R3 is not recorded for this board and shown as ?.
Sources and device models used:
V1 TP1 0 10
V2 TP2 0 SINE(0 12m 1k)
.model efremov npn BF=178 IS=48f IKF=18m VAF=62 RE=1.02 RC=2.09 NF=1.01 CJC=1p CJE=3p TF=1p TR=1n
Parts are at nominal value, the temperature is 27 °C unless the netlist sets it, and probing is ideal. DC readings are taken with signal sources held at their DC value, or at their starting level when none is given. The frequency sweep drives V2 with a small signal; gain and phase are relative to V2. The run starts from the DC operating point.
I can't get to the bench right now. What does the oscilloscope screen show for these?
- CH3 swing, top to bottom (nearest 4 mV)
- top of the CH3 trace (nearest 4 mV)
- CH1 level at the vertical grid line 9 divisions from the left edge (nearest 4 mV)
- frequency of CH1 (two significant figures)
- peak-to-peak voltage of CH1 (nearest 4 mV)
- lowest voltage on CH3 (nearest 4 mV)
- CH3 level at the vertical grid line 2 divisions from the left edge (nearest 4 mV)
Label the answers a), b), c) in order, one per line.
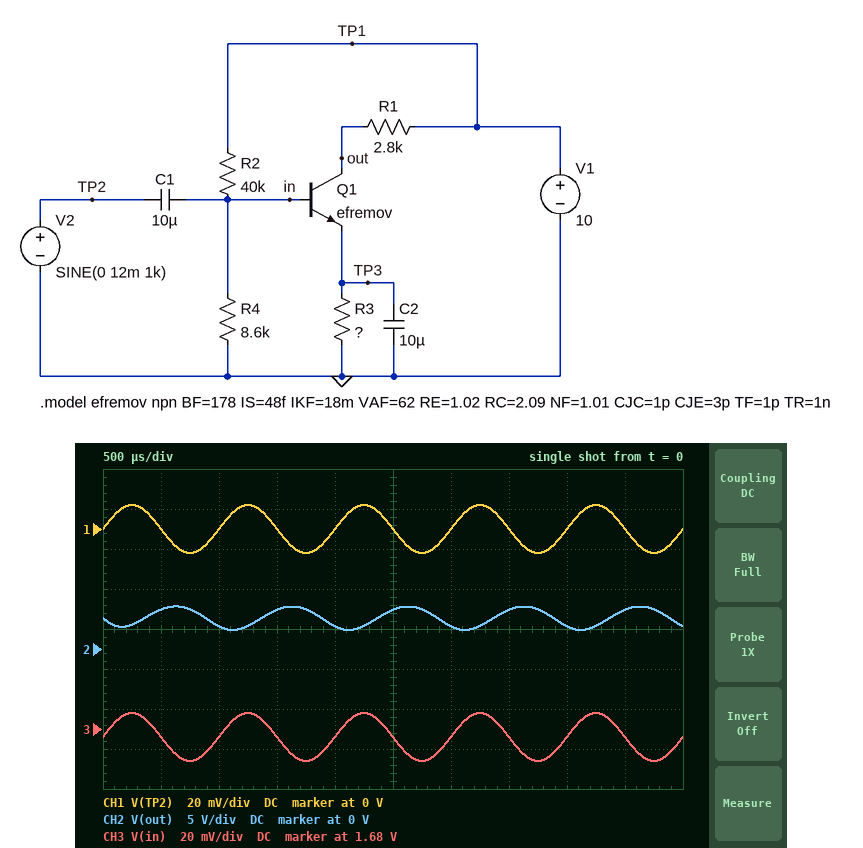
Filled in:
a) 24 mV
b) 1.688 V
c) 0 V
d) 1.0 kHz
e) 24 mV
f) 1.664 V
g) 1.676 V
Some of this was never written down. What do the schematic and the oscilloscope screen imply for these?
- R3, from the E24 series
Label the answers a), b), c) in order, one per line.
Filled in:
a) 470 Ω
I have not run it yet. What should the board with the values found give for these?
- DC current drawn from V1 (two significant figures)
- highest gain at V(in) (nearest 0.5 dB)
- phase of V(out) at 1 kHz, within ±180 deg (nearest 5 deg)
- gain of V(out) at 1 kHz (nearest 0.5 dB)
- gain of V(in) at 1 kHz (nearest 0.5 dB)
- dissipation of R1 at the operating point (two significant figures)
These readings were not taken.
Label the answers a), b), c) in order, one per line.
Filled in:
a) 2.4 mA
b) 0 dB
c) -135 deg
d) 42.0 dB
e) 0 dB
f) 13 mW
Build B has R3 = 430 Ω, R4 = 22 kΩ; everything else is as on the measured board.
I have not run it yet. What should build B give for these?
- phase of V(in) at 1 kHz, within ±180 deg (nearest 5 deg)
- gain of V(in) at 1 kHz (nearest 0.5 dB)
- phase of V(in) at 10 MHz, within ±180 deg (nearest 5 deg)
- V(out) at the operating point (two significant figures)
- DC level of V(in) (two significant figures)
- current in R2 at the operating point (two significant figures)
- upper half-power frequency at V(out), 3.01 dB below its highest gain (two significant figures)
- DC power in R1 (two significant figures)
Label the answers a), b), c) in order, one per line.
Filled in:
a) 20 deg
b) -3.5 dB
c) 0 deg
d) 1.5 V
e) 2.0 V
f) 200 µA
g) 210 MHz
h) 26 mW
